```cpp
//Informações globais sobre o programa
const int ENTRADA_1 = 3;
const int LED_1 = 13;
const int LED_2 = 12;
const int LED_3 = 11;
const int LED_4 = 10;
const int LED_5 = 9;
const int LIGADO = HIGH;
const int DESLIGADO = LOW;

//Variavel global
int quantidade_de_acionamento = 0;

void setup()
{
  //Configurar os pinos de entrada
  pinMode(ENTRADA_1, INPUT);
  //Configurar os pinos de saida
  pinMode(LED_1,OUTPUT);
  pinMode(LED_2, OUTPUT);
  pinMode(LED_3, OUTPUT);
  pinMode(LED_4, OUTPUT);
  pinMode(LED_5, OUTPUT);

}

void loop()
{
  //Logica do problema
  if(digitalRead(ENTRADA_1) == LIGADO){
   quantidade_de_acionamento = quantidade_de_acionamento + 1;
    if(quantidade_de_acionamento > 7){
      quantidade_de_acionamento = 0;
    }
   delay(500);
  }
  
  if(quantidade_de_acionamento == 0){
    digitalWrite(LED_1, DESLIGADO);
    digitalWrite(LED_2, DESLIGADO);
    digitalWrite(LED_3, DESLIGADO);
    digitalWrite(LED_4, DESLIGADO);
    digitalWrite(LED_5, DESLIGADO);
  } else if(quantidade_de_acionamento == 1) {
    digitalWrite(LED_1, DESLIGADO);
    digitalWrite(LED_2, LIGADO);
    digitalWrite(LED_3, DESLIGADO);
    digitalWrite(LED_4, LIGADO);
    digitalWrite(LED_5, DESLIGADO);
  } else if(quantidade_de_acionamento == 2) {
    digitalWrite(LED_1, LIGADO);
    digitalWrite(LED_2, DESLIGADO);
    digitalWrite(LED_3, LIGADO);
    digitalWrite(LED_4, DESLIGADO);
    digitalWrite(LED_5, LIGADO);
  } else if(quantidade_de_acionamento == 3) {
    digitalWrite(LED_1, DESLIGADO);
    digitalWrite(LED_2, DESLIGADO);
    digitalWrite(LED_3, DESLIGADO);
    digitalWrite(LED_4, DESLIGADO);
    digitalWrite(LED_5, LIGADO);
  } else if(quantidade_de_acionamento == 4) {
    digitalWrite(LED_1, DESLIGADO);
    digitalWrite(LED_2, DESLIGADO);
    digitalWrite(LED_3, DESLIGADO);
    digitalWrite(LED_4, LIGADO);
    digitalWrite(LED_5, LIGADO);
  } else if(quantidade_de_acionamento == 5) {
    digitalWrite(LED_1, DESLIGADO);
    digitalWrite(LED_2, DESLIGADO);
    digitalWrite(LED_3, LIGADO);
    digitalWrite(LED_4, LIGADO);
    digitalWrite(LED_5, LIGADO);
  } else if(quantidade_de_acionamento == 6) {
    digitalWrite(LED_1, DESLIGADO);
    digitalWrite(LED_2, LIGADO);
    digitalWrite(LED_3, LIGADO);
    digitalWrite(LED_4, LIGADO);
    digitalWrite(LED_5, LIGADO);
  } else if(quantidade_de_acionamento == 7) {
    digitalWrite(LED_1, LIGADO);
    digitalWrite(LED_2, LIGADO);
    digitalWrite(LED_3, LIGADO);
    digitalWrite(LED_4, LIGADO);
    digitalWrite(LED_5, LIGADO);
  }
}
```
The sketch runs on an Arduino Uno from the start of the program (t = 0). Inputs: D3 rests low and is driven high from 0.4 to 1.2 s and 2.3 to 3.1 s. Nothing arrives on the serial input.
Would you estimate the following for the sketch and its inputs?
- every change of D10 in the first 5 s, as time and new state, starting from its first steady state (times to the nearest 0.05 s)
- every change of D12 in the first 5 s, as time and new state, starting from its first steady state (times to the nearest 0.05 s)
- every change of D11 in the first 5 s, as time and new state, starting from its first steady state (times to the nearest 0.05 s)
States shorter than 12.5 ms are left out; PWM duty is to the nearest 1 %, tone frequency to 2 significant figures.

0 s low; 0.9 s high; 1.4 s low; 3.3 s high
0 s low; 0.9 s high; 1.4 s low
0 s low; 1.4 s high; 2.8 s low
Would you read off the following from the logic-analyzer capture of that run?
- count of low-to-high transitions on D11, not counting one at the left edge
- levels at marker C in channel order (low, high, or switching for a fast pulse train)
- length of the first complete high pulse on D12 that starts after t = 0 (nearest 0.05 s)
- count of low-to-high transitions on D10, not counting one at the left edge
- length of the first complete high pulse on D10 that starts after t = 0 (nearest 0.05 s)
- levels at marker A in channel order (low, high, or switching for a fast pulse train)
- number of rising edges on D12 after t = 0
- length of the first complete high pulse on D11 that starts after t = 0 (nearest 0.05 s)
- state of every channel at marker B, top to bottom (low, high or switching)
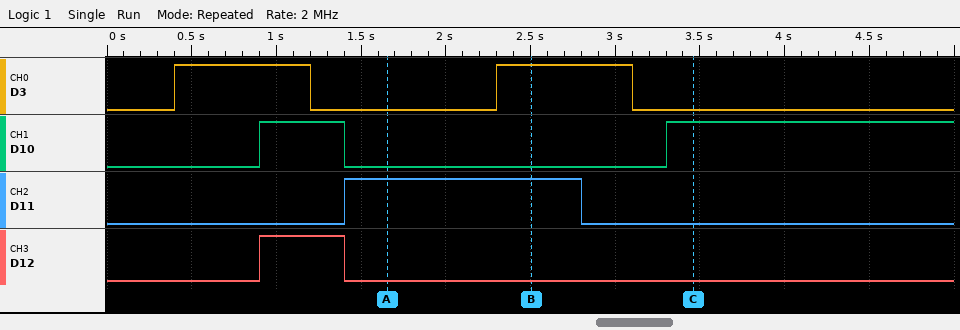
1
D3 low, D10 high, D11 low, D12 low
0.50 s
2
0.50 s
D3 low, D10 low, D11 high, D12 low
1
1.40 s
D3 high, D10 low, D11 high, D12 low
